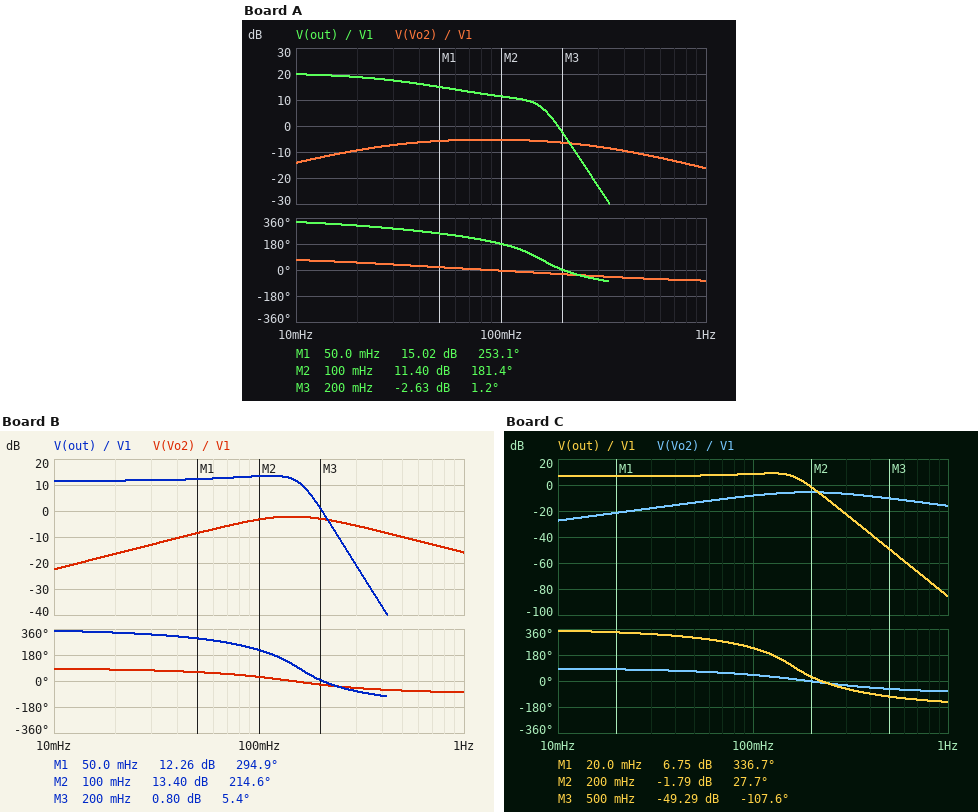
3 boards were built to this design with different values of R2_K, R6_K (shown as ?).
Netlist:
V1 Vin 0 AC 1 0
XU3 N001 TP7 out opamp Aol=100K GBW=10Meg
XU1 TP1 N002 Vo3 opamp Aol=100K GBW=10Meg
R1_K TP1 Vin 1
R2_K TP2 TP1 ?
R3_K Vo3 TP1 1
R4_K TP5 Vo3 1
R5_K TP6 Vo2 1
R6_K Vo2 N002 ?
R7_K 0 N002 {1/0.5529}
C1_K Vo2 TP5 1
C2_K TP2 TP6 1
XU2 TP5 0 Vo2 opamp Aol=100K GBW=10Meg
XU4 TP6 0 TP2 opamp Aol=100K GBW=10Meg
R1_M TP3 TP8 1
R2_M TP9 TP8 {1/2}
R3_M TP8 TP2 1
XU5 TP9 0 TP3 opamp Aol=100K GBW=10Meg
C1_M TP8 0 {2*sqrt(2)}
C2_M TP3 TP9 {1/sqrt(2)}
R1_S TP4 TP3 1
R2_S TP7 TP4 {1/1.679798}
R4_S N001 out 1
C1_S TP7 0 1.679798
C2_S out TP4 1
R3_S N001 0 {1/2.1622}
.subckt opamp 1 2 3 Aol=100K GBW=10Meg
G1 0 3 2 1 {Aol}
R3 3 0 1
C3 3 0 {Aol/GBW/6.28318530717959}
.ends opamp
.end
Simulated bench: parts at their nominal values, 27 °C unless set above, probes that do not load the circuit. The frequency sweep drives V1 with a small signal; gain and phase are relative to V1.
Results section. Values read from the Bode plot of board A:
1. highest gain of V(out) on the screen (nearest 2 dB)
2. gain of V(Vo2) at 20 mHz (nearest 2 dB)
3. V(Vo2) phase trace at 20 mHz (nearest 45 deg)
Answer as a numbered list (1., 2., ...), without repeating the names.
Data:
1. 20 dB
2. -10 dB
3. 45 deg
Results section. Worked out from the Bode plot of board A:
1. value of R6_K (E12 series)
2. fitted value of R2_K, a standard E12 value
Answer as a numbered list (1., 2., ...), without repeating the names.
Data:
1. 0.47 Ω
2. 3.3 Ω
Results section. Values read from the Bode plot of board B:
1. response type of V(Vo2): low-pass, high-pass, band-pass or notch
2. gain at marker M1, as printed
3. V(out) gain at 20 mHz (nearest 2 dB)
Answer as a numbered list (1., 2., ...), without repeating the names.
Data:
1. band-pass
2. 12.26 dB
3. 12 dB
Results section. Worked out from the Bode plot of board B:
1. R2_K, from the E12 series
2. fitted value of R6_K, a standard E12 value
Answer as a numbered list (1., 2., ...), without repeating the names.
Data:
1. 1.2 Ω
2. 2.2 Ω
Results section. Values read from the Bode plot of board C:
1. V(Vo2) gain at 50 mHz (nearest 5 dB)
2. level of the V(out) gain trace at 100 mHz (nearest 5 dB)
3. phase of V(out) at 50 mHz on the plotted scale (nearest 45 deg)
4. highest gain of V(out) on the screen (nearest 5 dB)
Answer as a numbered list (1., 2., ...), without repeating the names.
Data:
1. -15 dB
2. 10 dB
3. 315 deg
4. 10 dB
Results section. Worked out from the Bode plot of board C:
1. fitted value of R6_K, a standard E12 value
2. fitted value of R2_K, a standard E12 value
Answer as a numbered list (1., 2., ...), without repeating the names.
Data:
1. 1.5 Ω
2. 0.68 Ω
